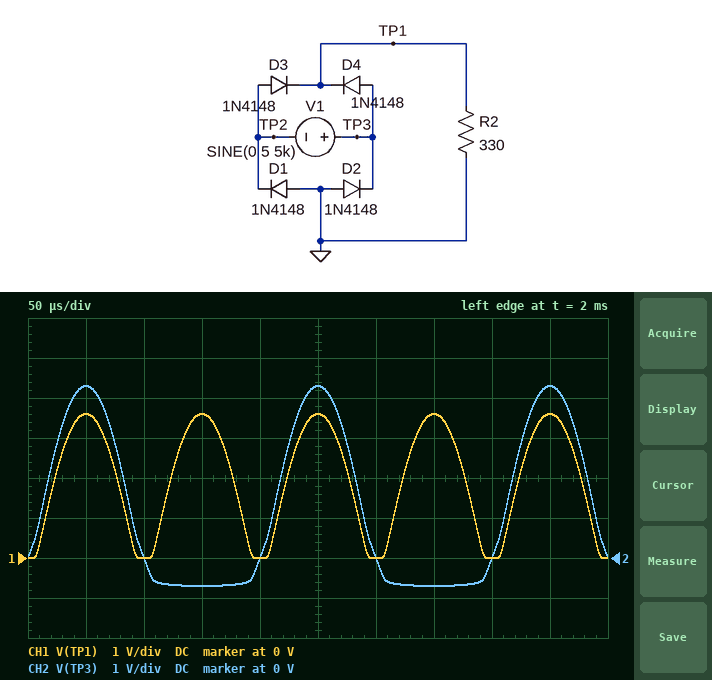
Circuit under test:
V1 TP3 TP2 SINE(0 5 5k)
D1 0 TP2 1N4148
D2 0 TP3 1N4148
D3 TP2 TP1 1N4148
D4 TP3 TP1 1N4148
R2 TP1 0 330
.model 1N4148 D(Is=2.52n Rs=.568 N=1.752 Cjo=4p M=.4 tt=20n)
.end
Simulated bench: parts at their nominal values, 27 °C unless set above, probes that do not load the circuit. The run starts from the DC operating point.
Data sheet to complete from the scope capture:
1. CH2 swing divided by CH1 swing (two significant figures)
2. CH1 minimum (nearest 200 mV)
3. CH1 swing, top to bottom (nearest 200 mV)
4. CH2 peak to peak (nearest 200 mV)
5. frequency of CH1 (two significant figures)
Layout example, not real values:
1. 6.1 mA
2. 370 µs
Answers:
1. 1.4
2. 0 V
3. 3.6 V
4. 5.0 V
5. 10 kHz
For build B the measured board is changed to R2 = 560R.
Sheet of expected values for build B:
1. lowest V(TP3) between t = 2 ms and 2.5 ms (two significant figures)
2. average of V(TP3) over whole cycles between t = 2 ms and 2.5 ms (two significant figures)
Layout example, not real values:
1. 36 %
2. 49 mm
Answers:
1. -670 mV
2. 1.0 V
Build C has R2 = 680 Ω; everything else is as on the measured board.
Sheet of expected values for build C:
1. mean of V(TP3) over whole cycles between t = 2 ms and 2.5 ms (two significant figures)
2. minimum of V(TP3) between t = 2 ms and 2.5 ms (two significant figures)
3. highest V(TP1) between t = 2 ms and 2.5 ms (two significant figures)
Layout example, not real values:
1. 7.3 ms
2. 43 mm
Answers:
1. 1.0 V
2. -660 mV
3. 3.7 V
